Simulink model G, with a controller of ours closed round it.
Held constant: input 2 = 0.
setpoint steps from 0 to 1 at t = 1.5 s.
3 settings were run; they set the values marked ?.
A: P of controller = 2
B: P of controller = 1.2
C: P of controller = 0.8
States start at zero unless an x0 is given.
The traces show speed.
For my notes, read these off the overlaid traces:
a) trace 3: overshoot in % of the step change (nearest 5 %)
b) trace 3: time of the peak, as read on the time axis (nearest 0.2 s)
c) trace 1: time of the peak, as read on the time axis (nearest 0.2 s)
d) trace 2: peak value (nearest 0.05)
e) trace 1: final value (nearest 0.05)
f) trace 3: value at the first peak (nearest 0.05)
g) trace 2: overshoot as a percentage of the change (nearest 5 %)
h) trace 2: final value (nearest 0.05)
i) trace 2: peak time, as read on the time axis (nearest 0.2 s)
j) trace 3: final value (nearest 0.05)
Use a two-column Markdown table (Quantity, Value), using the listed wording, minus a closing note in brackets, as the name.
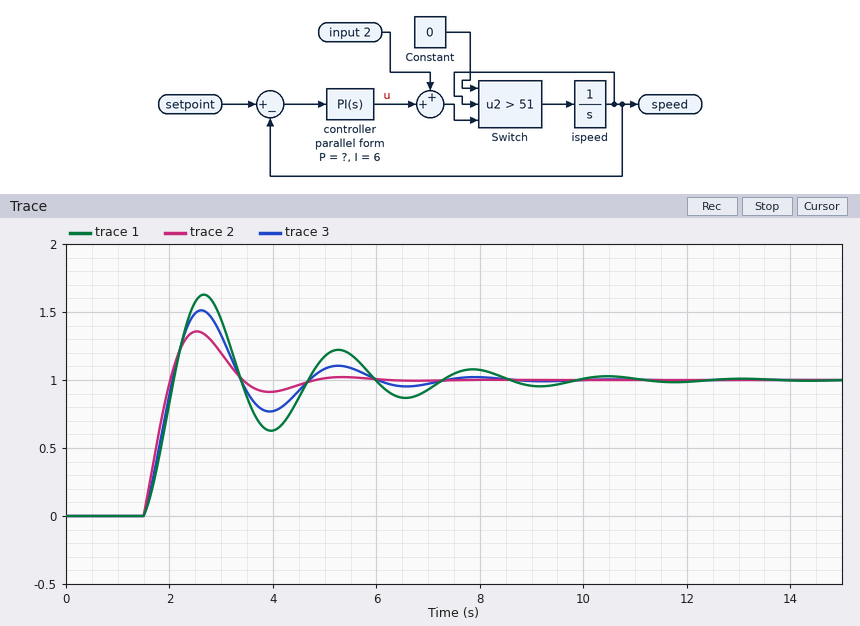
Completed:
| Quantity | Value |
|---|---|
| trace 3: overshoot in % of the step change | 50 % |
| trace 3: time of the peak, as read on the time axis | 2.6 s |
| trace 1: time of the peak, as read on the time axis | 2.6 s |
| trace 2: peak value | 1.35 |
| trace 1: final value | 1.00 |
| trace 3: value at the first peak | 1.50 |
| trace 2: overshoot as a percentage of the change | 35 % |
| trace 2: final value | 1.00 |
| trace 2: peak time, as read on the time axis | 2.6 s |
| trace 3: final value | 1.00 |
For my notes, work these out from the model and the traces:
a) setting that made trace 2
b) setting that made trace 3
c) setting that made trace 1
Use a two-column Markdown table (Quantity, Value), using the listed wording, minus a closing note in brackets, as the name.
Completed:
| Quantity | Value |
|---|---|
| setting that made trace 2 | A |
| setting that made trace 3 | B |
| setting that made trace 1 | C |
